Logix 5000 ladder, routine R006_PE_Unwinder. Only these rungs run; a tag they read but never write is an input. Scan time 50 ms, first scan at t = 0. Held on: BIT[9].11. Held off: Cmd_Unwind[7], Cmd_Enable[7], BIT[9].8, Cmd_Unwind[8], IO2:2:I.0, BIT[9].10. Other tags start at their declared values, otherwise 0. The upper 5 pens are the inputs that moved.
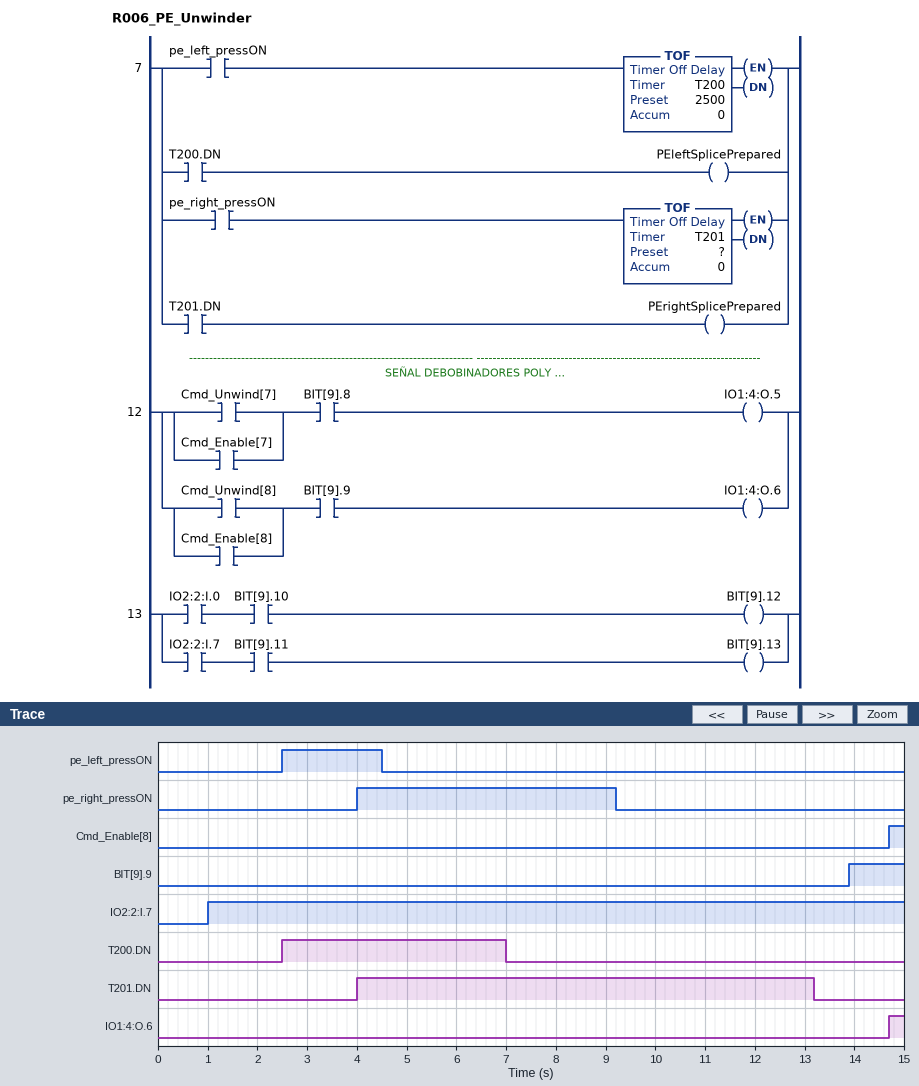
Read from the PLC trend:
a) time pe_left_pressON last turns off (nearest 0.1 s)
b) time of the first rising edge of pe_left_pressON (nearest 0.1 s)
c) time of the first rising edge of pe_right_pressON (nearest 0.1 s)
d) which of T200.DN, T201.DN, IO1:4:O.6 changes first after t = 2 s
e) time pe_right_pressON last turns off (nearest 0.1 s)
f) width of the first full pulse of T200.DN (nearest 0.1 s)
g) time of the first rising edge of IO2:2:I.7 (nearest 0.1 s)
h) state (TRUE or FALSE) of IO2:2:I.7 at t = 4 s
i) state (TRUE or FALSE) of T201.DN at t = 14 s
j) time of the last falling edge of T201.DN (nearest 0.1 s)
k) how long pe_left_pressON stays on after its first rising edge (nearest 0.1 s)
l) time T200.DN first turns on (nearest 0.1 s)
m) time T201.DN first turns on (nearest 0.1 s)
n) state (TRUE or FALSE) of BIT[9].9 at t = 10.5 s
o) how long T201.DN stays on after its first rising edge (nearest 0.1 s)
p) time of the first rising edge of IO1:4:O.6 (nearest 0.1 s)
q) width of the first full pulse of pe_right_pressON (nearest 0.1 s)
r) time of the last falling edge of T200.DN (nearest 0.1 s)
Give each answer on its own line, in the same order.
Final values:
4.5 s
2.5 s
4.0 s
T200.DN
9.2 s
4.5 s
1.0 s
TRUE
FALSE
13.2 s
2.0 s
2.5 s
4.0 s
FALSE
9.2 s
14.7 s
5.2 s
7.0 s
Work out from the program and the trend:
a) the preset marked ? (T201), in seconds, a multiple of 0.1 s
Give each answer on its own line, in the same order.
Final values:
4.0 s
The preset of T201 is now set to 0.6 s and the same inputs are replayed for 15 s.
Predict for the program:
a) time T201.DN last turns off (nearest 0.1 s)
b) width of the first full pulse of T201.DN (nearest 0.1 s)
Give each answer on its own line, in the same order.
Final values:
9.8 s
5.8 s
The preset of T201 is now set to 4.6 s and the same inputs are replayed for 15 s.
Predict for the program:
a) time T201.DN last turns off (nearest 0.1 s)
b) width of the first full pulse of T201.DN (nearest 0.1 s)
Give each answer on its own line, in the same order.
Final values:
13.8 s
9.8 s
